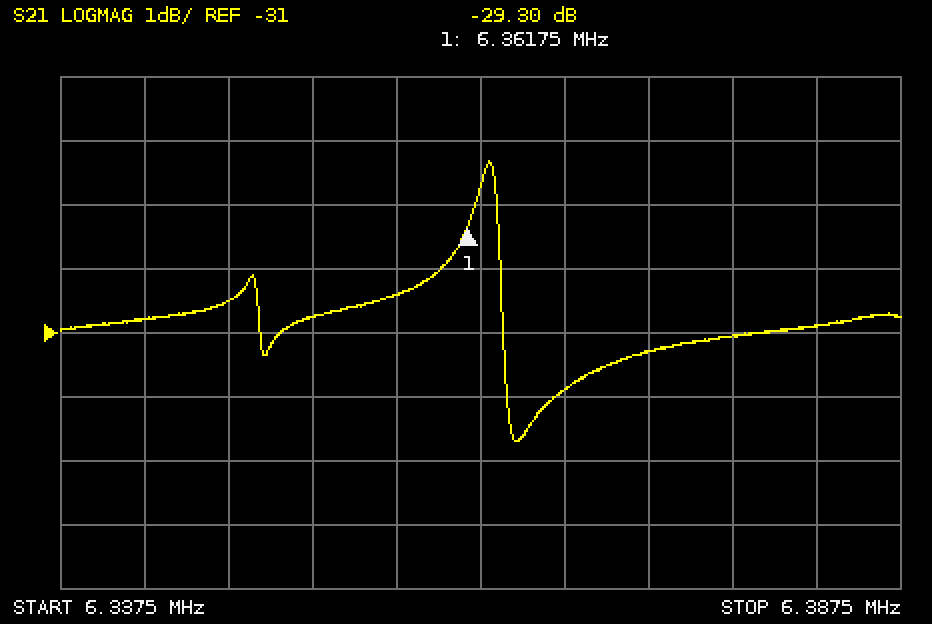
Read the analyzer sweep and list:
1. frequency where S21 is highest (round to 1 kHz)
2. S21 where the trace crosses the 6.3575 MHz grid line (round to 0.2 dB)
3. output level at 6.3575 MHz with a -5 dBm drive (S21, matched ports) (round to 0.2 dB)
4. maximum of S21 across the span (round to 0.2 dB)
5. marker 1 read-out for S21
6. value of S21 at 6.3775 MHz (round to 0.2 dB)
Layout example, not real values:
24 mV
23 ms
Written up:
6.363 MHz
-30.4 dB
-35.4 dBm
-28.4 dB
-29.30 dB
-31.0 dB
